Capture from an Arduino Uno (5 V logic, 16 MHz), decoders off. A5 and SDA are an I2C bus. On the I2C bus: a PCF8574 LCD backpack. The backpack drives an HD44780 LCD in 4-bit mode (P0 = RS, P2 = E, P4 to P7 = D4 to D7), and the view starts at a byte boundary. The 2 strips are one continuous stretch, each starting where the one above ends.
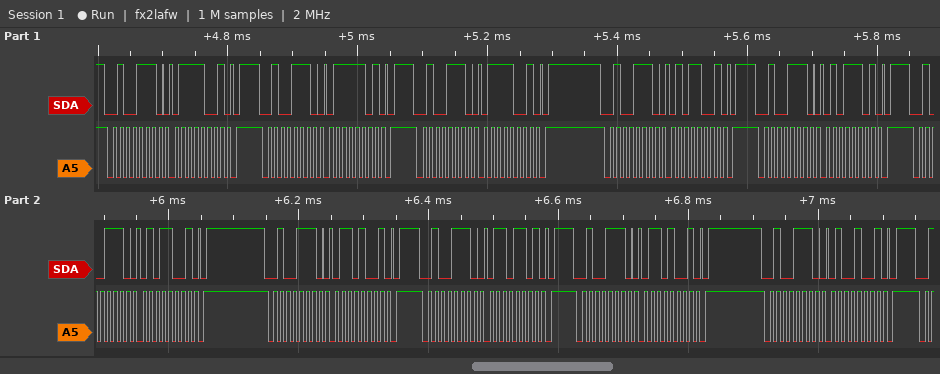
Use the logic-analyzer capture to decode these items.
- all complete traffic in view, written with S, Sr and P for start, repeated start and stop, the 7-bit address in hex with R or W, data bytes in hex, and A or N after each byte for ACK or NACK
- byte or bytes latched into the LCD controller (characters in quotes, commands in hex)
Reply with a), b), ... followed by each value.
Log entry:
a) S 27W A 79 A P S 27W A 7D A P S 27W A 79 A P S 27W A 59 A P S 27W A 5D A P S 27W A 59 A P S 27W A 69 A P S 27W A 6D A P S 27W A 69 A P S 27W A 49 A P
b) 'u'
